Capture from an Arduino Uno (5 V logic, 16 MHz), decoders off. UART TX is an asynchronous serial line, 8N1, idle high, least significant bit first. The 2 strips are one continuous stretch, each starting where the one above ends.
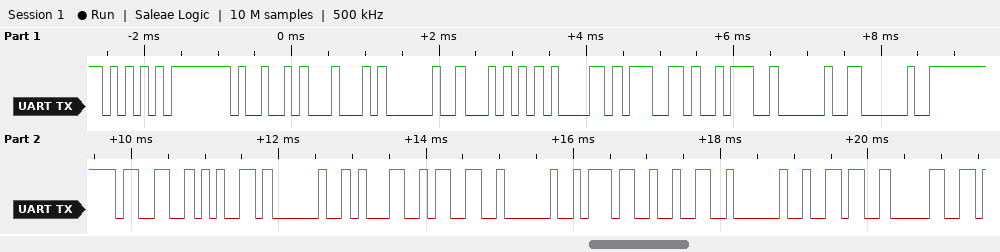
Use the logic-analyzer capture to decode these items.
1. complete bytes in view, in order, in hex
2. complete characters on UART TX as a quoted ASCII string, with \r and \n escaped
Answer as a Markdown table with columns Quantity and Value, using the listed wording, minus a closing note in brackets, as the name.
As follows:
| Quantity | Value |
|---|---|
| complete bytes in view, in order, in hex | 0x55 0x49 0x44 0x20 0x54 0x61 0x67 0x3A 0x20 0x20 0x33 0x65 0x20 0x31 0x33 0x20 0x37 0x32 0x20 0x36 0x30 |
| complete characters on UART TX as a quoted ASCII string, with \r and \n escaped | "UID Tag:  3e 13 72 60" |
